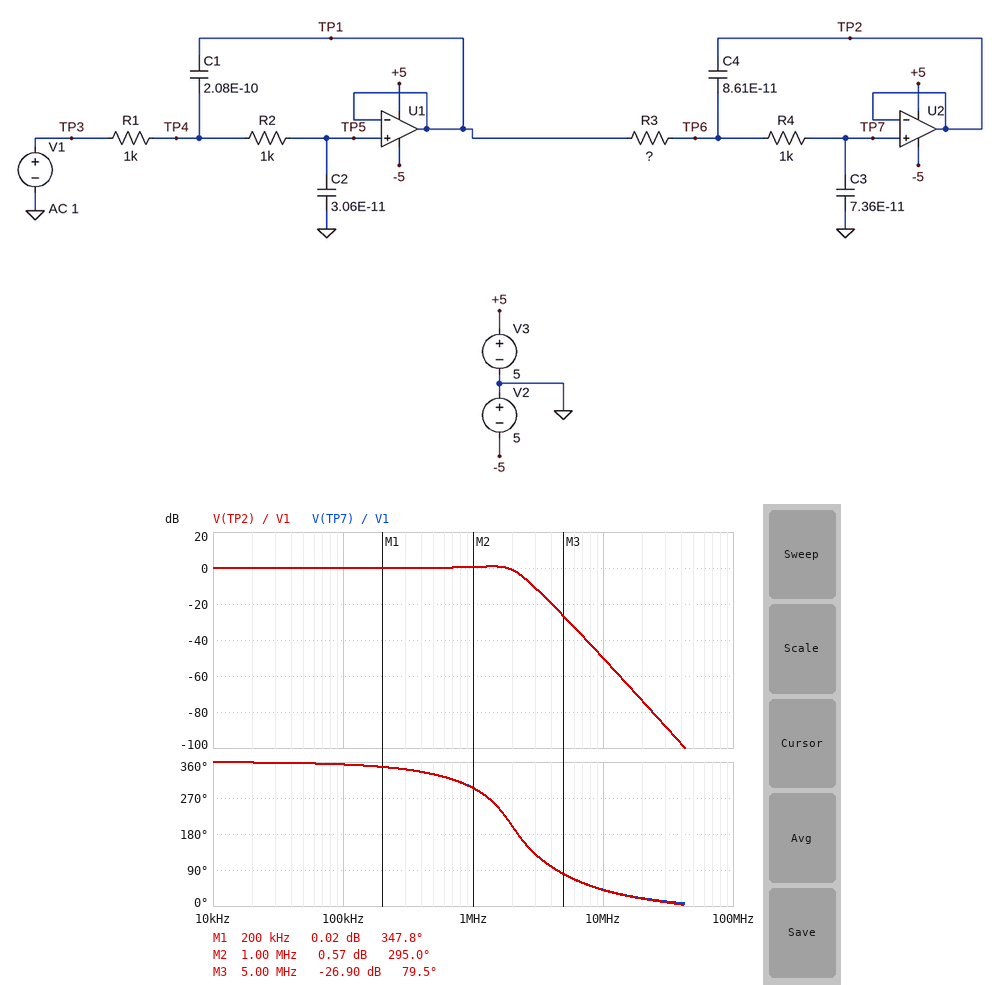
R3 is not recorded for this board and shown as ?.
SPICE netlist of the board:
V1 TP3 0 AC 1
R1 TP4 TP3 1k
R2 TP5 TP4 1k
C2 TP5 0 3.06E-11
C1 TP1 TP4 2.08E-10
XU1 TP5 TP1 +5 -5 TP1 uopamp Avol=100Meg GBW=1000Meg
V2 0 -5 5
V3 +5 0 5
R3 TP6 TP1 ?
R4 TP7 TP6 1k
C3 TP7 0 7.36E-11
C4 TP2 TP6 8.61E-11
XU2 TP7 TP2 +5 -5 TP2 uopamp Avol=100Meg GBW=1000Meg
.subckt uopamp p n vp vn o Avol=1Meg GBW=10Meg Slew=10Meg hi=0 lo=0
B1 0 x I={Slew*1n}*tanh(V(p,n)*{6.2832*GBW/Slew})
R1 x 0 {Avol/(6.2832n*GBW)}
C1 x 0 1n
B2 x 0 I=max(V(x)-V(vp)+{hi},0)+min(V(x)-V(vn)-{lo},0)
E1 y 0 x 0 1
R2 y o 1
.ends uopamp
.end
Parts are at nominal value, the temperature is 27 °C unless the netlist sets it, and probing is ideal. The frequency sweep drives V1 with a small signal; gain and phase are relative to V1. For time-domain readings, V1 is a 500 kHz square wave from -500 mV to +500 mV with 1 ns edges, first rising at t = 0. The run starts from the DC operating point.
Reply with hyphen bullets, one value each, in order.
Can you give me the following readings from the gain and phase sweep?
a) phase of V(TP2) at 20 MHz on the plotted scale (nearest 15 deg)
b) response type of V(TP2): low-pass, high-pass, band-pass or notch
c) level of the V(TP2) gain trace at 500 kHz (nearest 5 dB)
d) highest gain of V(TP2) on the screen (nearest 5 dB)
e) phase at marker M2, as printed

- 15 deg
- low-pass
- 0 dB
- 0 dB
- 295.0 deg
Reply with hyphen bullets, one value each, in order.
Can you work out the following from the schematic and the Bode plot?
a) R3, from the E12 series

- 470 Ω
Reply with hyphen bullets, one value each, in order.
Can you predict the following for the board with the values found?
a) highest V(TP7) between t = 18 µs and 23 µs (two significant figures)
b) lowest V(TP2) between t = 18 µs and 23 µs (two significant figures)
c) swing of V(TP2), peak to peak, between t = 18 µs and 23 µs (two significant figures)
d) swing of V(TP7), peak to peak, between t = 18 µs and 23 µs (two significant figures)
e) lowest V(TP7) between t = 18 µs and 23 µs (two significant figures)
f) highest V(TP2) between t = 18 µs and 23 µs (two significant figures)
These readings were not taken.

- 660 mV
- -660 mV
- 1.3 V
- 1.3 V
- -660 mV
- 660 mV
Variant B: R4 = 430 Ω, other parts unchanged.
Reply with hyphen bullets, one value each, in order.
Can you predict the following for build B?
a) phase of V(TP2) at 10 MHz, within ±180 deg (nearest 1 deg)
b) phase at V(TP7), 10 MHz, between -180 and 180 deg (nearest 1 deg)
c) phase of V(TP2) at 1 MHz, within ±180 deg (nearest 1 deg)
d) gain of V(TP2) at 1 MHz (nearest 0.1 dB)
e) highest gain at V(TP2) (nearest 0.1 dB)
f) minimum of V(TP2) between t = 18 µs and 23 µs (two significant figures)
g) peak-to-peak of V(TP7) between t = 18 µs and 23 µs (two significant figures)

- 53 deg
- 54 deg
- -51 deg
- 1.2 dB
- 2.2 dB
- -730 mV
- 1.5 V
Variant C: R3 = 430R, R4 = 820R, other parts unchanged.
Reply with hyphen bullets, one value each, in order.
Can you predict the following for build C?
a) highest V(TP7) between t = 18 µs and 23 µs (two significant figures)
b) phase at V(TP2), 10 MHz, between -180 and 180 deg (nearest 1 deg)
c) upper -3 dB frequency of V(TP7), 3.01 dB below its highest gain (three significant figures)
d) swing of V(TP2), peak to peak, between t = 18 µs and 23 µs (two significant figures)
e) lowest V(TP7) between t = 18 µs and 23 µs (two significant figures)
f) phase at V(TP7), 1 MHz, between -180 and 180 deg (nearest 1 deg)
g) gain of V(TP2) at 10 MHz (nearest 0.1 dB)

- 690 mV
- 44 deg
- 2.19 MHz
- 1.4 V
- -690 mV
- -60 deg
- -47.6 dB
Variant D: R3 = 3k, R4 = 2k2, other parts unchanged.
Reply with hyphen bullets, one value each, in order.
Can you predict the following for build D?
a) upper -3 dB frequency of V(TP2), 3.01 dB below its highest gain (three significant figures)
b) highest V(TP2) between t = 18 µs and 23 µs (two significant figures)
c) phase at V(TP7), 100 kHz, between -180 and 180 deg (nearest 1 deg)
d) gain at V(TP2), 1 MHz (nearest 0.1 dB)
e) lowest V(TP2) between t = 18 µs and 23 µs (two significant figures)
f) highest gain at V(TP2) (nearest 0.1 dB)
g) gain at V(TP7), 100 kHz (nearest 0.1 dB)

- 606 kHz
- 480 mV
- -16 deg
- -6.4 dB
- -480 mV
- 0 dB
- -0.1 dB
